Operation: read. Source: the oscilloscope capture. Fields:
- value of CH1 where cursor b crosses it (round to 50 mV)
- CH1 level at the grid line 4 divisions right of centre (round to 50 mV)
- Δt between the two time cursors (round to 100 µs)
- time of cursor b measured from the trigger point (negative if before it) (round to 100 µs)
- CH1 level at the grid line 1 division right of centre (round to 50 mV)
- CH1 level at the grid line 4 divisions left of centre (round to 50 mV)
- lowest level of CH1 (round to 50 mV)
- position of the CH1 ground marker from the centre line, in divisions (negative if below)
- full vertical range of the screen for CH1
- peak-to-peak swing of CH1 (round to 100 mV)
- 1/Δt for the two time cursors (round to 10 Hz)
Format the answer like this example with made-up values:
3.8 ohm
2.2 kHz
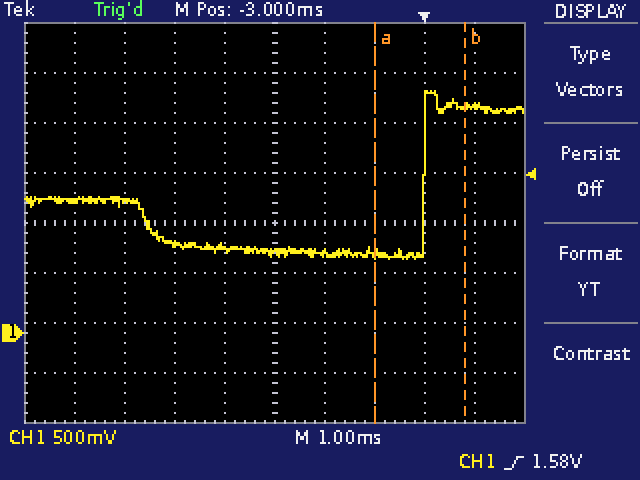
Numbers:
2.25 V
2.25 V
1.8 ms
+800 µs
800 mV
1.30 V
750 mV
-2.2 div
4 V
1.70 V
560 Hz
